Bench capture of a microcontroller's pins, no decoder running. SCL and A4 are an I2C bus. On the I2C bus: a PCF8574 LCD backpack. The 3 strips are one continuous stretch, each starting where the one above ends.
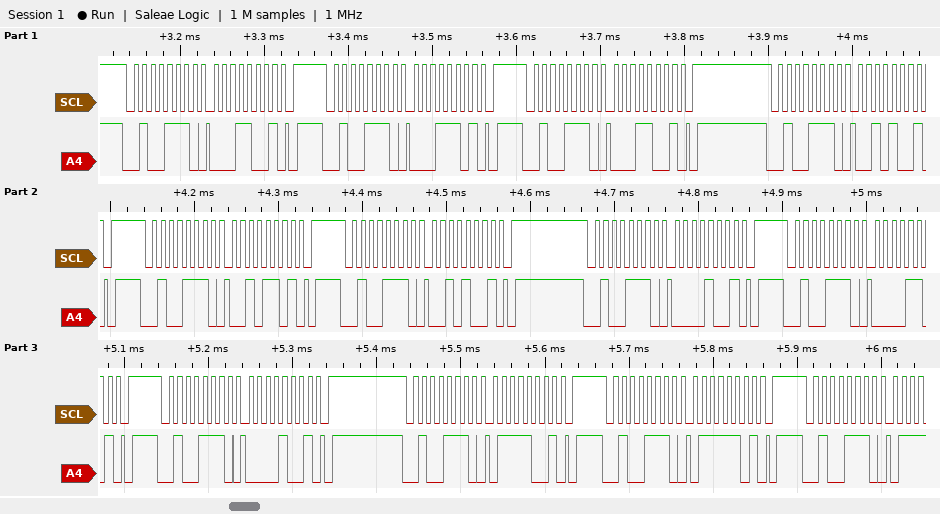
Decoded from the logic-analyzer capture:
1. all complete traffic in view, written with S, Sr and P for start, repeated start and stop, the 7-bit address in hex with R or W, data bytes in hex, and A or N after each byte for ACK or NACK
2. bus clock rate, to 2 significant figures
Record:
S 27W A 19 A P S 27W A 1D A P S 27W A 19 A P S 27W A 29 A P S 27W A 2D A P S 27W A 29 A P S 27W A 09 A P S 27W A 0D A P S 27W A 09 A P S 27W A 79 A P S 27W A 7D A P S 27W A
100 kHz
